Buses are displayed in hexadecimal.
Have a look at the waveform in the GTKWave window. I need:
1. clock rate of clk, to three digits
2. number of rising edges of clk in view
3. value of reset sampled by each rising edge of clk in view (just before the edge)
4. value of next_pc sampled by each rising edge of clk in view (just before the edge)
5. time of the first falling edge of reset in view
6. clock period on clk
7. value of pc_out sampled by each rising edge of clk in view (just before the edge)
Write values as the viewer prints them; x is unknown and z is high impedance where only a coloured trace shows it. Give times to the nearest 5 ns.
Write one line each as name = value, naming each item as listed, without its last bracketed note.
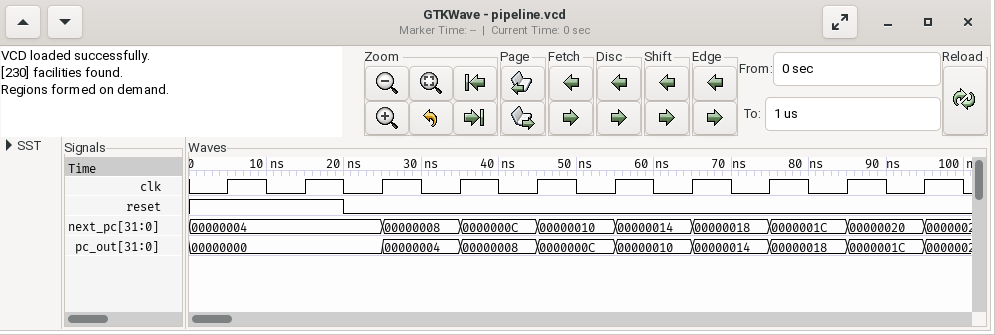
clock rate of clk, to three digits = 100 MHz
number of rising edges of clk in view = 10
value of reset sampled by each rising edge of clk in view = 1 1 0 0 0 0 0 0 0 0
value of next_pc sampled by each rising edge of clk in view = 00000004, 00000004, 00000004, 00000008, 0000000C, 00000010, 00000014, 00000018, 0000001C, 00000020
time of the first falling edge of reset in view = 20 ns
clock period on clk = 10 ns
value of pc_out sampled by each rising edge of clk in view = 00000000, 00000000, 00000000, 00000004, 00000008, 0000000C, 00000010, 00000014, 00000018, 0000001C
